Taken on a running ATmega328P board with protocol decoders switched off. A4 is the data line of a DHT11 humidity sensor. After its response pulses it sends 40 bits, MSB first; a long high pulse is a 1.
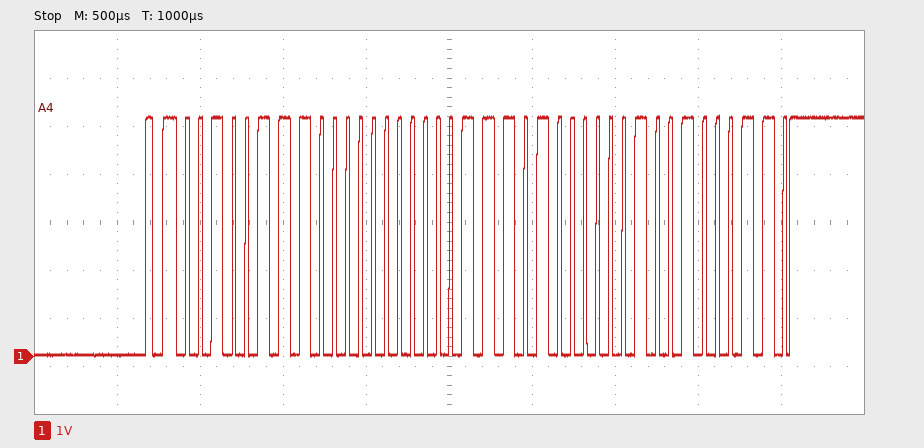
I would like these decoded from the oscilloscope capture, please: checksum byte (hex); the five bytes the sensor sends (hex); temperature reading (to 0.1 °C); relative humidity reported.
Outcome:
0x46
27 00 1D 02 46
29.2 °C
39 %
